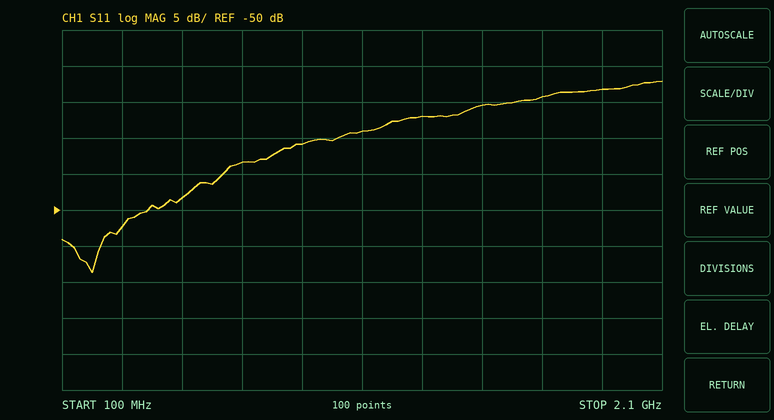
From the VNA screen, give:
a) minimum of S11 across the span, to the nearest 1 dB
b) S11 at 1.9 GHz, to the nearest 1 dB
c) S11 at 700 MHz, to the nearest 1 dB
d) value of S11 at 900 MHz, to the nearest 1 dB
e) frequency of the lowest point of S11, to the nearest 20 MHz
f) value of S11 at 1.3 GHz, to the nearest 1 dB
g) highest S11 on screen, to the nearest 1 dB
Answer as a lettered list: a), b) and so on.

a) -59 dB
b) -33 dB
c) -43 dB
d) -41 dB
e) 200 MHz
f) -37 dB
g) -32 dB
